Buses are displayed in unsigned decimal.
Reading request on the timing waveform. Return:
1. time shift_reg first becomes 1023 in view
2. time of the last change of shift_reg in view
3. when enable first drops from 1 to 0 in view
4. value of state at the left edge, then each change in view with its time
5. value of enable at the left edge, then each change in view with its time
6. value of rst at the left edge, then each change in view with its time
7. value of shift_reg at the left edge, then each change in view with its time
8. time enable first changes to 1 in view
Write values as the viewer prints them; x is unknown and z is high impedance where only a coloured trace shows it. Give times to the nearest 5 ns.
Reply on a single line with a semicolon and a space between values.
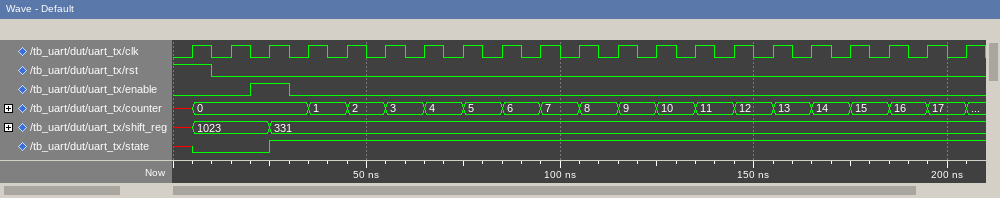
5 ns; 25 ns; 30 ns; x, 0 at 5 ns, 1 at 25 ns; 0, 1 at 20 ns, 0 at 30 ns; 1, 0 at 10 ns; x, 1023 at 5 ns, 331 at 25 ns; 20 ns
